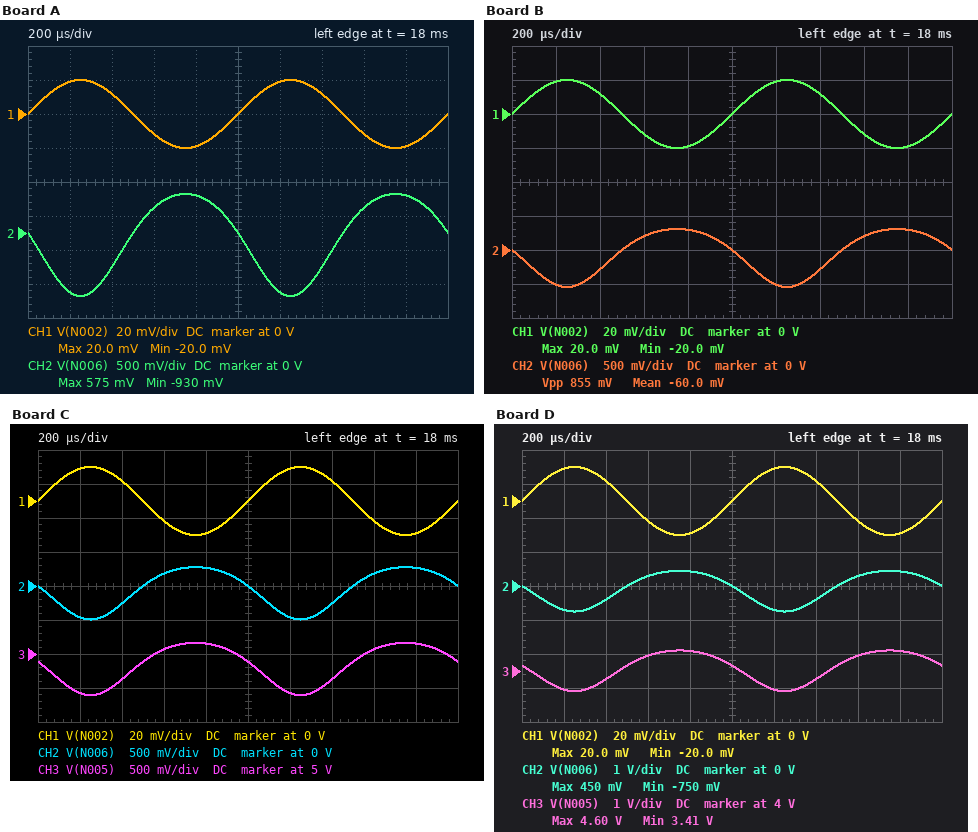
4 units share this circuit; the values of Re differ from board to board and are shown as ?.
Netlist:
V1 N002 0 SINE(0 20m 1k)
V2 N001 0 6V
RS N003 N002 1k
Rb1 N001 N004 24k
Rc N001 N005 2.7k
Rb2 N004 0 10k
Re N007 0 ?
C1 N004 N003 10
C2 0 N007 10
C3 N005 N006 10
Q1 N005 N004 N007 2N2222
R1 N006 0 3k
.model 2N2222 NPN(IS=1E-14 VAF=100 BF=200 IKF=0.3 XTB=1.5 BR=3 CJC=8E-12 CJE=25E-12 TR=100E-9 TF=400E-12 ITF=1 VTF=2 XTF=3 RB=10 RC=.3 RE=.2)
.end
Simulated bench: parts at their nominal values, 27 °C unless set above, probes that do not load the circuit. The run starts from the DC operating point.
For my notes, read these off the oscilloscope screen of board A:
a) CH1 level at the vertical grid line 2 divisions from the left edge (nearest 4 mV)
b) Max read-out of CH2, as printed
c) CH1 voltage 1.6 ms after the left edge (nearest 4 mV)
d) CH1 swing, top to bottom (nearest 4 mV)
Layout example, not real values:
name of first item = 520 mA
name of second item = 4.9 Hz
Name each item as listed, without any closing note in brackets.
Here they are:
CH1 level at the vertical grid line 2 divisions from the left edge = 12 mV
Max read-out of CH2, as printed = 575 mV
CH1 voltage 1.6 ms after the left edge = -12 mV
CH1 swing, top to bottom = 40 mV
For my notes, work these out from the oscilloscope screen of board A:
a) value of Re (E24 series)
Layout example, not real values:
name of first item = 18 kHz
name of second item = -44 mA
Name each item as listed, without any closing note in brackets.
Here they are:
value of Re = 1.2 kΩ
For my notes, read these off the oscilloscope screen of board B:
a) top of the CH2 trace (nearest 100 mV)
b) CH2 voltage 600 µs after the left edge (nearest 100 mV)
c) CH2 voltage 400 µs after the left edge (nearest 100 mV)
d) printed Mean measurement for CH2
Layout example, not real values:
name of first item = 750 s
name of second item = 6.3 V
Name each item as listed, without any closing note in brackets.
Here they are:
top of the CH2 trace = 300 mV
CH2 voltage 600 µs after the left edge = 200 mV
CH2 voltage 400 µs after the left edge = -300 mV
printed Mean measurement for CH2 = -60.0 mV
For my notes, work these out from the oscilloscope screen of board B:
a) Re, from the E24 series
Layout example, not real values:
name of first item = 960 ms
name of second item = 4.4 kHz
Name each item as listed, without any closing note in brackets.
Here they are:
Re, from the E24 series = 2.4 kΩ
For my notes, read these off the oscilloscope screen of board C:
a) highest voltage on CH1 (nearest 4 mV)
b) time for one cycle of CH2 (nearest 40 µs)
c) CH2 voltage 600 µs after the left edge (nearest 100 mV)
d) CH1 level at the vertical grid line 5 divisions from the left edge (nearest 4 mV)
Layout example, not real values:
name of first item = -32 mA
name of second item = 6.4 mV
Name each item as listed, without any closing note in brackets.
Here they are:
highest voltage on CH1 = 20 mV
time for one cycle of CH2 = 1.00 ms
CH2 voltage 600 µs after the left edge = 200 mV
CH1 level at the vertical grid line 5 divisions from the left edge = 0 V
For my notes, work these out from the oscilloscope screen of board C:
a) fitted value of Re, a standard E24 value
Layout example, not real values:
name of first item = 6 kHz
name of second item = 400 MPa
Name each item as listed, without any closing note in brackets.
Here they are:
fitted value of Re, a standard E24 value = 2.7 kΩ
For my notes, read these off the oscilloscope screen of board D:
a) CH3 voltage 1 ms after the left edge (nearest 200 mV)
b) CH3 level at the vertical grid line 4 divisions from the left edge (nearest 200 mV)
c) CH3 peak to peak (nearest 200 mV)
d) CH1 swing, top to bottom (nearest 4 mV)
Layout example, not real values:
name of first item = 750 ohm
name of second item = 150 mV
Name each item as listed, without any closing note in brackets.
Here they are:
CH3 voltage 1 ms after the left edge = 4.2 V
CH3 level at the vertical grid line 4 divisions from the left edge = 4.6 V
CH3 peak to peak = 1.2 V
CH1 swing, top to bottom = 40 mV
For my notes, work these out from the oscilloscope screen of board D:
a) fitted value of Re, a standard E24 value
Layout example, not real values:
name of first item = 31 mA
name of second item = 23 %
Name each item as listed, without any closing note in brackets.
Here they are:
fitted value of Re, a standard E24 value = 1.6 kΩ
